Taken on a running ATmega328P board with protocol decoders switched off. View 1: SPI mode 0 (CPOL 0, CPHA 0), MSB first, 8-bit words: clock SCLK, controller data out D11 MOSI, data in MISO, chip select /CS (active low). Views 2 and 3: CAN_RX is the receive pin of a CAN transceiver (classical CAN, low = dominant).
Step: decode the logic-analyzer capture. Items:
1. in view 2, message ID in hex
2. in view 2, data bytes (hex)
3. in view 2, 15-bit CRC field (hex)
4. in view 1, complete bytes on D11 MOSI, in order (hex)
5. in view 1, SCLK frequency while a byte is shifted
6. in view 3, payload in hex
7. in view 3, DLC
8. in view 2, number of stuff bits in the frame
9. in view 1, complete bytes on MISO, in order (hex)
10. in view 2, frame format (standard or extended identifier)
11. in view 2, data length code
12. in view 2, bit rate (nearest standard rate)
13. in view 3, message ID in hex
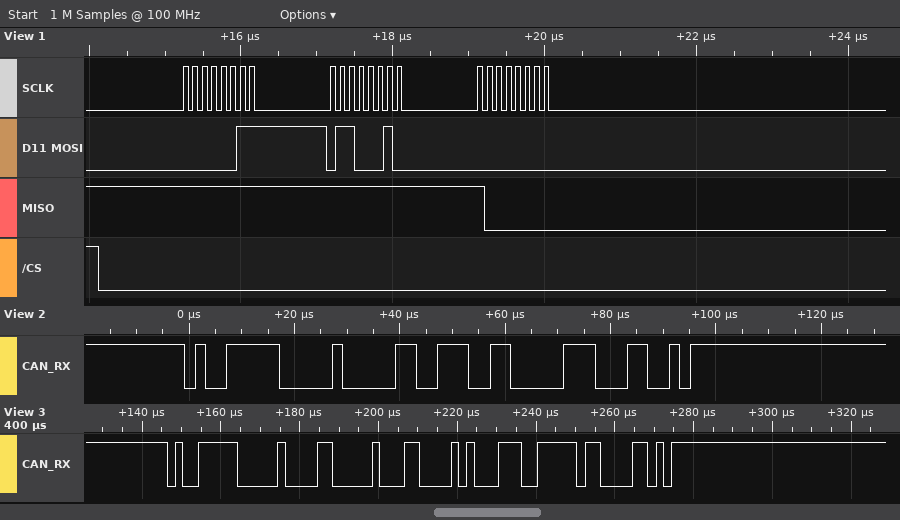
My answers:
0x4F8
39
0x418C
03 62 00
8 MHz
00 C2 8E
3
4
FF FF 80
standard
1
500 kbit/s
0x4F8
